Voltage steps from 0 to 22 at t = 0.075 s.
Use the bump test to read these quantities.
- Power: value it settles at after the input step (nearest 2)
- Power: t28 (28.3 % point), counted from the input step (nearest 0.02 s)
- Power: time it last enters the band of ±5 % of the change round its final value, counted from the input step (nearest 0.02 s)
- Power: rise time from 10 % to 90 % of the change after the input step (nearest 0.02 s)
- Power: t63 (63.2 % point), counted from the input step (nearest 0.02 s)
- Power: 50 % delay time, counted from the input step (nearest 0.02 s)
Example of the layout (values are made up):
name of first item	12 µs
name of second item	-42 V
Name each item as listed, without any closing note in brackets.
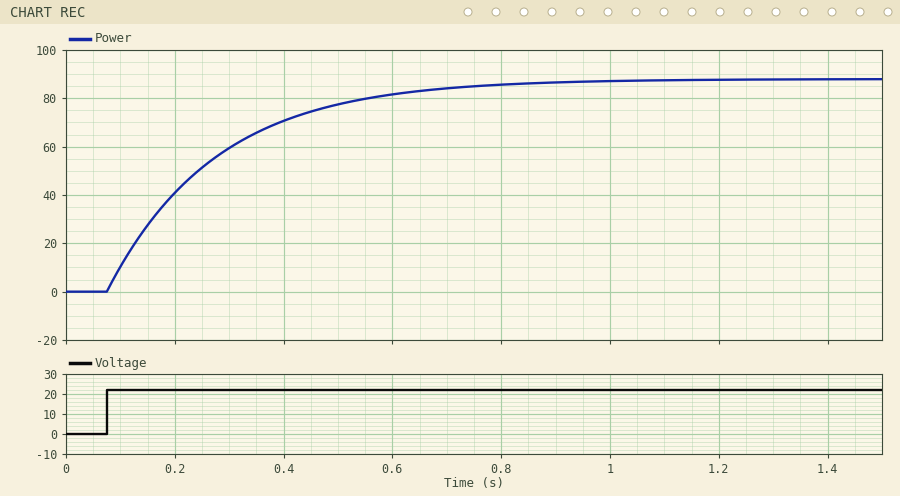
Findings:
Power: value it settles at after the input step	88
Power: t28 (28.3 % point), counted from the input step	0.06 s
Power: time it last enters the band of ±5 % of the change round its final value, counted from the input step	0.60 s
Power: rise time from 10 % to 90 % of the change after the input step	0.44 s
Power: t63 (63.2 % point), counted from the input step	0.20 s
Power: 50 % delay time, counted from the input step	0.14 s
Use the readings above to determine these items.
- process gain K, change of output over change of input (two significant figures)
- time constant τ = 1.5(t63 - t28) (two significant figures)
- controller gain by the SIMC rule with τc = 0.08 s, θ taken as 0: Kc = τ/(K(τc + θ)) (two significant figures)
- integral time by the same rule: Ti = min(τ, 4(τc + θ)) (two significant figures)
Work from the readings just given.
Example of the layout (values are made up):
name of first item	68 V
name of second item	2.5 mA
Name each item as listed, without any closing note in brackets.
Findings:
process gain K, change of output over change of input	4.0
time constant τ = 1.5(t63 - t28)	0.21 s
controller gain by the SIMC rule with τc = 0.08 s, θ taken as 0: Kc = τ/(K(τc + θ))	0.66
integral time by the same rule: Ti = min(τ, 4(τc + θ))	0.21 s
